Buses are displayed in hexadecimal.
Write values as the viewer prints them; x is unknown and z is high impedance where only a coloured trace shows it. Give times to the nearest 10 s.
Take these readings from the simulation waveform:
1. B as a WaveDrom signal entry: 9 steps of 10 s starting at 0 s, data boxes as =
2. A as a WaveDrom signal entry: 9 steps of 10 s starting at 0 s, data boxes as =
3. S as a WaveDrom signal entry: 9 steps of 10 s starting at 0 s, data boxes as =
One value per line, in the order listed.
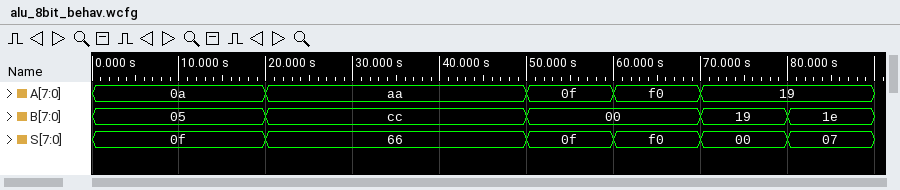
{name: 'B', wave: '=.=..=.==', data: '05 cc 00 19 1e'}
{name: 'A', wave: '=.=..===.', data: '0a aa 0f f0 19'}
{name: 'S', wave: '=.=..====', data: '0f 66 0f f0 00 07'}
